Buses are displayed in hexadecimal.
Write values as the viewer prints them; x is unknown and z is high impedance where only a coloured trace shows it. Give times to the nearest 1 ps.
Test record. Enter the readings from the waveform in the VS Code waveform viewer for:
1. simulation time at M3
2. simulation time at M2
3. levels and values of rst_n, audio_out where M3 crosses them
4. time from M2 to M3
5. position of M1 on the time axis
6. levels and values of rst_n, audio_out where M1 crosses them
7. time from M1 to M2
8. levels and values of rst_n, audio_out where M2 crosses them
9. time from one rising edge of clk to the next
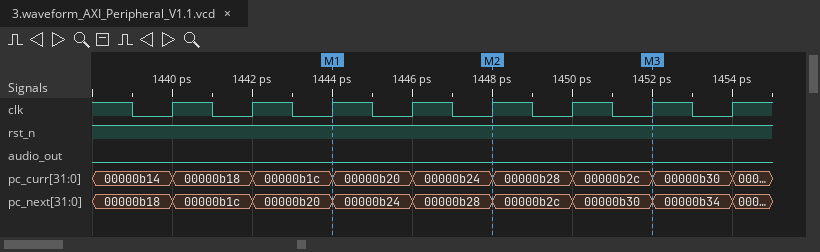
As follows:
1452 ps
1448 ps
rst_n=1, audio_out=0
4 ps
1444 ps
rst_n=1, audio_out=0
4 ps
rst_n=1, audio_out=0
2 ps
